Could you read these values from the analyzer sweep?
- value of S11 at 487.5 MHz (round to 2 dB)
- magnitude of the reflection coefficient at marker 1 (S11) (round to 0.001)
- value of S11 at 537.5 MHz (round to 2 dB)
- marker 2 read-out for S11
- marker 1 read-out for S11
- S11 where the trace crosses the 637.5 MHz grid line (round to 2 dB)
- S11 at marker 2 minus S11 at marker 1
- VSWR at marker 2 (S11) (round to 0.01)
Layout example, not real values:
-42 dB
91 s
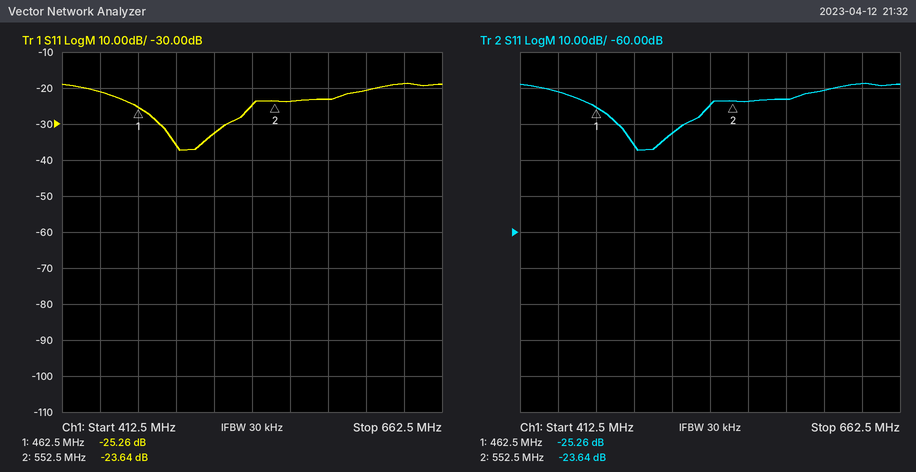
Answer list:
-36 dB
0.055
-24 dB
-23.64 dB
-25.26 dB
-18 dB
1.62 dB
1.14
